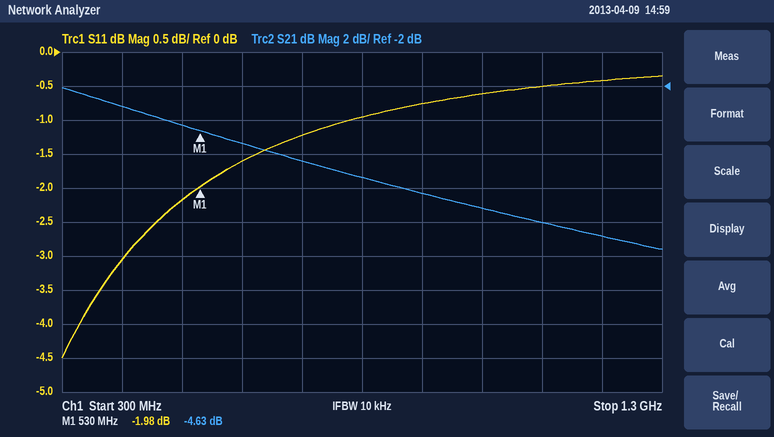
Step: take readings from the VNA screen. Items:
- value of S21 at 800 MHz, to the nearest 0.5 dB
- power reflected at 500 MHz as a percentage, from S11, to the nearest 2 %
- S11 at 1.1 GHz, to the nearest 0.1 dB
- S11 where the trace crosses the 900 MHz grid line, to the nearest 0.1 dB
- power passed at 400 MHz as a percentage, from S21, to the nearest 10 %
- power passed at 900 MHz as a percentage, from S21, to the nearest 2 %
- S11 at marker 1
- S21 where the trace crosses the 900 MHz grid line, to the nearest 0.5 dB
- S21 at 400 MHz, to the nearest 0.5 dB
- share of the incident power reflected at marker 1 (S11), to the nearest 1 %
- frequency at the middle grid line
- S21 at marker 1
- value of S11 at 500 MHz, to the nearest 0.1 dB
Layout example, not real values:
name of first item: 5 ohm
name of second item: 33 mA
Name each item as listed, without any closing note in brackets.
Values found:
value of S21 at 800 MHz, to the nearest 0.5 dB: -7.5 dB
power reflected at 500 MHz as a percentage, from S11, to the nearest 2 %: 60 %
S11 at 1.1 GHz, to the nearest 0.1 dB: -0.5 dB
S11 where the trace crosses the 900 MHz grid line, to the nearest 0.1 dB: -0.8 dB
power passed at 400 MHz as a percentage, from S21, to the nearest 10 %: 50 %
power passed at 900 MHz as a percentage, from S21, to the nearest 2 %: 14 %
S11 at marker 1: -1.98 dB
S21 where the trace crosses the 900 MHz grid line, to the nearest 0.5 dB: -8.5 dB
S21 at 400 MHz, to the nearest 0.5 dB: -3.0 dB
share of the incident power reflected at marker 1 (S11), to the nearest 1 %: 63 %
frequency at the middle grid line: 800 MHz
S21 at marker 1: -4.63 dB
value of S11 at 500 MHz, to the nearest 0.1 dB: -2.2 dB
